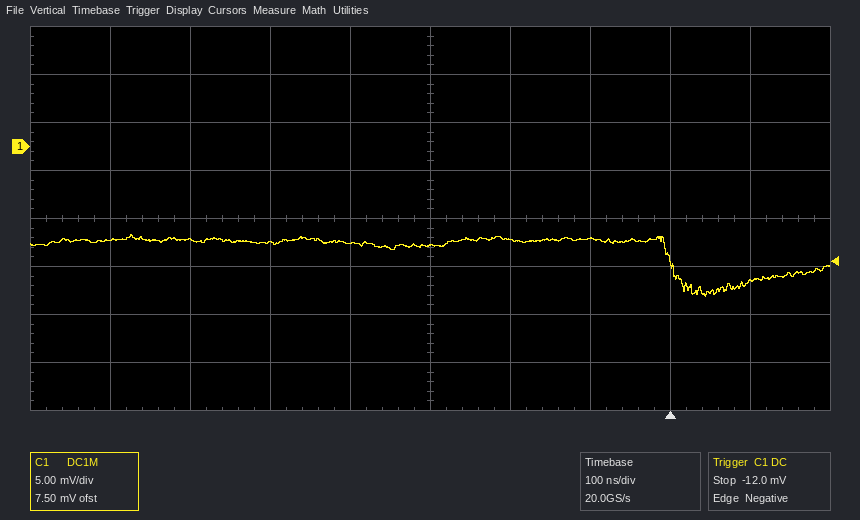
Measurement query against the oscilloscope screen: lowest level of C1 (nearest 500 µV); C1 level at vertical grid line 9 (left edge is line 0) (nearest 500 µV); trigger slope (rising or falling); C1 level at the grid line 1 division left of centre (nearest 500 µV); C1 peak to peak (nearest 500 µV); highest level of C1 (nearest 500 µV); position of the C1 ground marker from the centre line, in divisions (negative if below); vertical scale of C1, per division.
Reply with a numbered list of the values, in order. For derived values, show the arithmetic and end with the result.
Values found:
1. -15.5 mV
2. -14.0 mV
3. falling
4. -10.0 mV
5. -9.0 mV − (-15.5 mV) = 6.5 mV
6. -9.0 mV
7. +1.5 div
8. 5 mV
